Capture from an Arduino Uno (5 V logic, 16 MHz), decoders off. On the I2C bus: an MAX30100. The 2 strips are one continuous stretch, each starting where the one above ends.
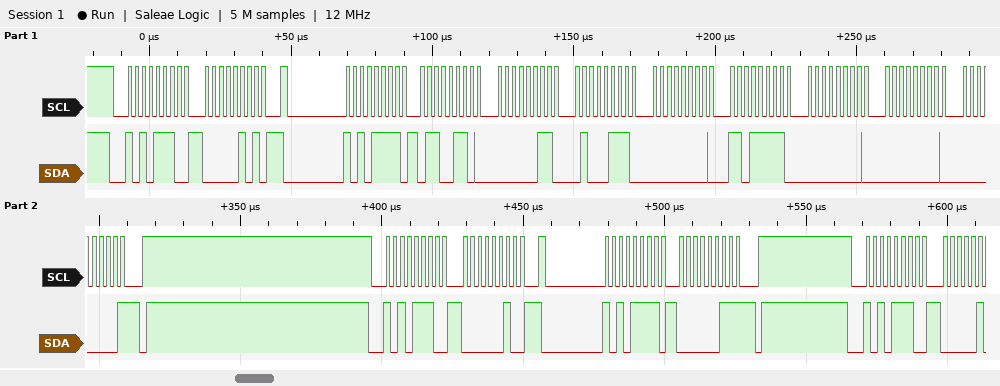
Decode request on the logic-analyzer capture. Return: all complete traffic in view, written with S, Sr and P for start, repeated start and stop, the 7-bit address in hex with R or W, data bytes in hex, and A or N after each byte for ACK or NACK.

S 57W A 05 A Sr 57R A 66 A 03 A 47 A 00 A DF A 00 A 00 A 00 N P S 57W A 02 A Sr 57R A 03 N P S 57W A
